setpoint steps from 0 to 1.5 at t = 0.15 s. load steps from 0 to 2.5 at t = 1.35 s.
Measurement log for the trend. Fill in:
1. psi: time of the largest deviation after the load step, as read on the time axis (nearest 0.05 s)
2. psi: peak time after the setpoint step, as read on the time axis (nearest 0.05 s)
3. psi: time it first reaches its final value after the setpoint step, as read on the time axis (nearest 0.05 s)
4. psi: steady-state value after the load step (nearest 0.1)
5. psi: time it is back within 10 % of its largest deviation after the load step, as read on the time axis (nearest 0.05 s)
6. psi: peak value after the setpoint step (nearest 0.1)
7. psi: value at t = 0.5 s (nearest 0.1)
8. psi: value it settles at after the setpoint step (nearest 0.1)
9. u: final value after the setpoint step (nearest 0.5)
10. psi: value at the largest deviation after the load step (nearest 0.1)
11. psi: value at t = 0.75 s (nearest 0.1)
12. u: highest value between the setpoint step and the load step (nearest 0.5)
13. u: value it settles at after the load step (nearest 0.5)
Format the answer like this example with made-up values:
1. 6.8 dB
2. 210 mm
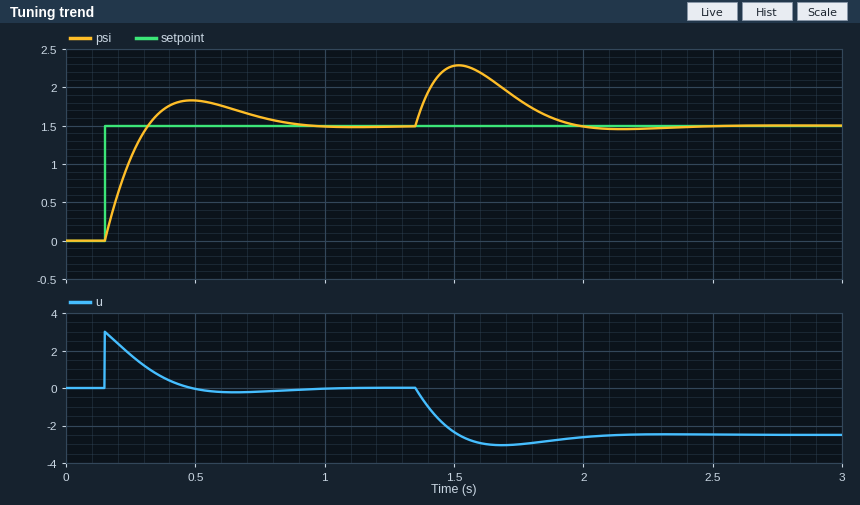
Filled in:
1. 1.50 s
2. 0.50 s
3. 0.30 s
4. 1.5
5. 1.90 s
6. 1.8
7. 1.8
8. 1.5
9. 0.0
10. 2.3
11. 1.6
12. 3.0
13. -2.5
